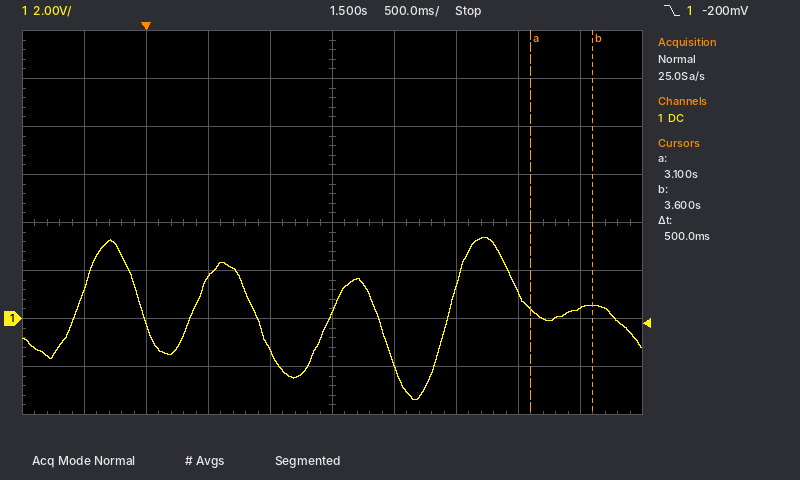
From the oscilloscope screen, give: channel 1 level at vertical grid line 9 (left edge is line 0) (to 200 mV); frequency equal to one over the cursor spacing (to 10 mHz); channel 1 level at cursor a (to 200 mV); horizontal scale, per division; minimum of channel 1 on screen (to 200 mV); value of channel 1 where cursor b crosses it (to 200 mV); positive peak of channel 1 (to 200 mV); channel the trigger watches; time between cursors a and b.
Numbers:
400 mV
2.00 Hz
400 mV
500 ms
-3.4 V
600 mV
3.4 V
channel 1
500 ms
